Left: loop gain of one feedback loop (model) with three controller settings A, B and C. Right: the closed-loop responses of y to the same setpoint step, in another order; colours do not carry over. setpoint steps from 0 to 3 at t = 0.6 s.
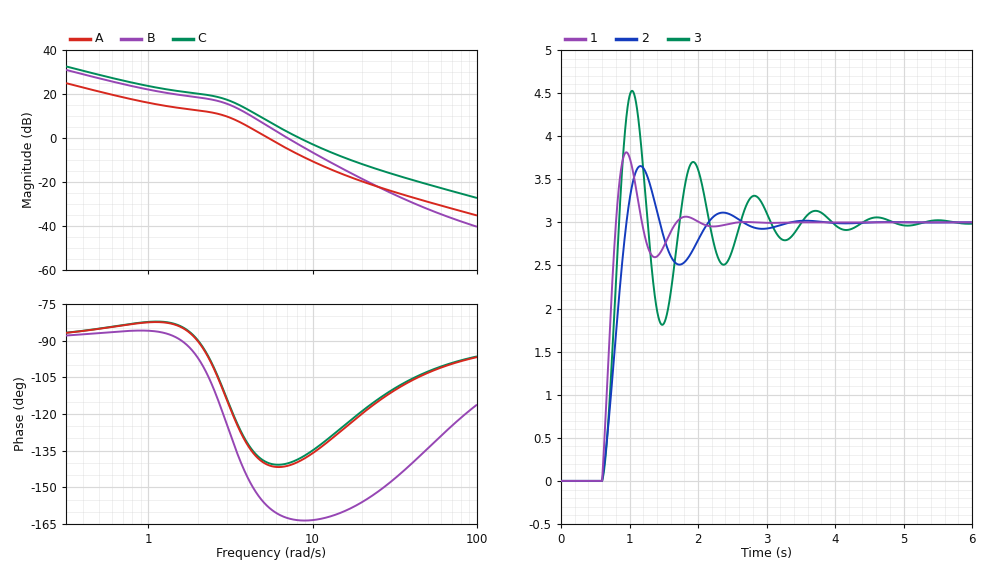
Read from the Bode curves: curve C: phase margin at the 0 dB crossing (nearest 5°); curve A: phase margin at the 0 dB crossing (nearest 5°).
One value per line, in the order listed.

40°
40°
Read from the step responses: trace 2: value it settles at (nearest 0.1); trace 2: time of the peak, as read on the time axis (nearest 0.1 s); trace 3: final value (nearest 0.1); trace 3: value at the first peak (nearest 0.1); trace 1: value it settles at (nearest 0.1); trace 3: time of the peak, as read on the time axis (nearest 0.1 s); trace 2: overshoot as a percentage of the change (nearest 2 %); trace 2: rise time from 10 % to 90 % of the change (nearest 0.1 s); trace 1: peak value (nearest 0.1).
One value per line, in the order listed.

3.0
1.2 s
3.0
4.5
3.0
1.0 s
22 %
0.3 s
3.8
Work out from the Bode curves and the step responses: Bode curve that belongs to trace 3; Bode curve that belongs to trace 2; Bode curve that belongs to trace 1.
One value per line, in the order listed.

B
A
C
